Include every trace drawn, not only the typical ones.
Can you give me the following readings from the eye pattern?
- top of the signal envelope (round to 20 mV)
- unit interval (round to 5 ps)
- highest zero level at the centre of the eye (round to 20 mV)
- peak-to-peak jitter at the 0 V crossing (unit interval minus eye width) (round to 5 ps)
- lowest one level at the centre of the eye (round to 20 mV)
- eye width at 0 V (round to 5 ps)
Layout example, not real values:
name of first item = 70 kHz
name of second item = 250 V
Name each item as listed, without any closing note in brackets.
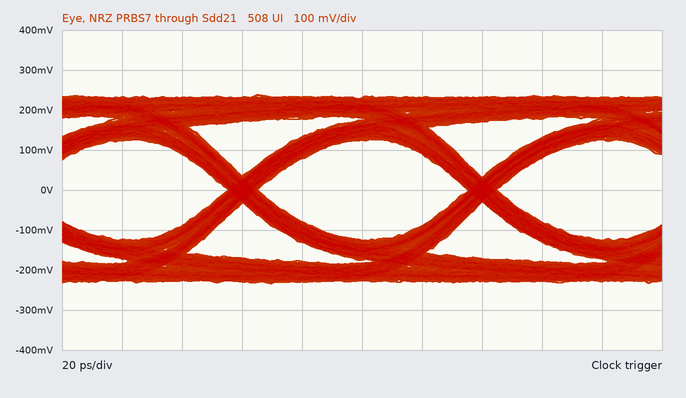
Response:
top of the signal envelope = 240 mV
unit interval = 80 ps
highest zero level at the centre of the eye = -120 mV
peak-to-peak jitter at the 0 V crossing (unit interval minus eye width) = 10 ps
lowest one level at the centre of the eye = 120 mV
eye width at 0 V = 70 ps
